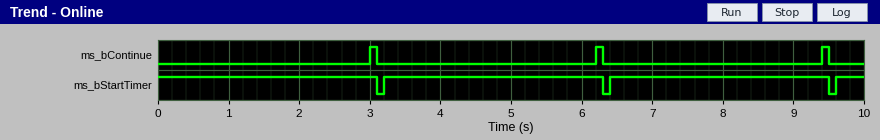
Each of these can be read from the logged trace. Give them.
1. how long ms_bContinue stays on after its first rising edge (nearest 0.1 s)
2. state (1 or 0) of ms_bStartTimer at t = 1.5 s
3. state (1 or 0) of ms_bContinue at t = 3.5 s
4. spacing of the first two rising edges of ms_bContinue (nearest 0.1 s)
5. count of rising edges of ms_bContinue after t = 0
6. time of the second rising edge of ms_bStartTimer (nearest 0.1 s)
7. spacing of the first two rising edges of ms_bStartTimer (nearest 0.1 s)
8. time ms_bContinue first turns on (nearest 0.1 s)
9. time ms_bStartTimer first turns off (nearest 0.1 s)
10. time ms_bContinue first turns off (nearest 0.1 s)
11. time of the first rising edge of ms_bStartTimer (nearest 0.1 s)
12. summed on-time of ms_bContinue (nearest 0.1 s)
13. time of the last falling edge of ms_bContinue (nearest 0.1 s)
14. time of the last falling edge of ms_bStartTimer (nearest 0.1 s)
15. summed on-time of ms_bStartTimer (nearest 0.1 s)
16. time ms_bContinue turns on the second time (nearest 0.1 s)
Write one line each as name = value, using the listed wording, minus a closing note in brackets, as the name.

how long ms_bContinue stays on after its first rising edge = 0.1 s
state (1 or 0) of ms_bStartTimer at t = 1.5 s = 1
state (1 or 0) of ms_bContinue at t = 3.5 s = 0
spacing of the first two rising edges of ms_bContinue = 3.2 s
count of rising edges of ms_bContinue after t = 0 = 3
time of the second rising edge of ms_bStartTimer = 6.4 s
spacing of the first two rising edges of ms_bStartTimer = 3.2 s
time ms_bContinue first turns on = 3.0 s
time ms_bStartTimer first turns off = 3.1 s
time ms_bContinue first turns off = 3.1 s
time of the first rising edge of ms_bStartTimer = 3.2 s
summed on-time of ms_bContinue = 0.3 s
time of the last falling edge of ms_bContinue = 9.5 s
time of the last falling edge of ms_bStartTimer = 9.5 s
summed on-time of ms_bStartTimer = 9.7 s
time ms_bContinue turns on the second time = 6.2 s
